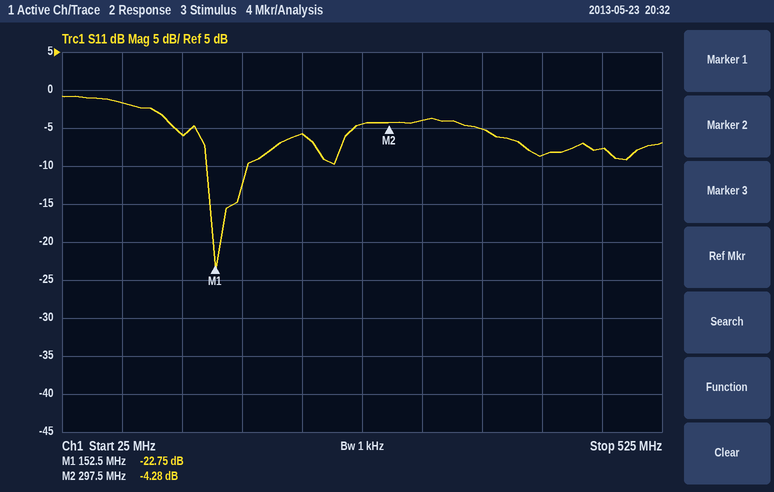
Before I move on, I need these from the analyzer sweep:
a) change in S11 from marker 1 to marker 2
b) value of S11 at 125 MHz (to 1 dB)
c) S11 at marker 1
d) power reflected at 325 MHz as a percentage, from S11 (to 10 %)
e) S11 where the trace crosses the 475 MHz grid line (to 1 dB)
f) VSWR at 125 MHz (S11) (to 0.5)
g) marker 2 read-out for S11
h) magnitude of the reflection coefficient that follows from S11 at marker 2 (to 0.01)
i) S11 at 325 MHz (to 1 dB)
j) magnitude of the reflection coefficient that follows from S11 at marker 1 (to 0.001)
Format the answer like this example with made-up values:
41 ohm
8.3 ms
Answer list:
18.47 dB
-6 dB
-22.75 dB
40 %
-8 dB
3.0
-4.28 dB
0.61
-4 dB
0.073
